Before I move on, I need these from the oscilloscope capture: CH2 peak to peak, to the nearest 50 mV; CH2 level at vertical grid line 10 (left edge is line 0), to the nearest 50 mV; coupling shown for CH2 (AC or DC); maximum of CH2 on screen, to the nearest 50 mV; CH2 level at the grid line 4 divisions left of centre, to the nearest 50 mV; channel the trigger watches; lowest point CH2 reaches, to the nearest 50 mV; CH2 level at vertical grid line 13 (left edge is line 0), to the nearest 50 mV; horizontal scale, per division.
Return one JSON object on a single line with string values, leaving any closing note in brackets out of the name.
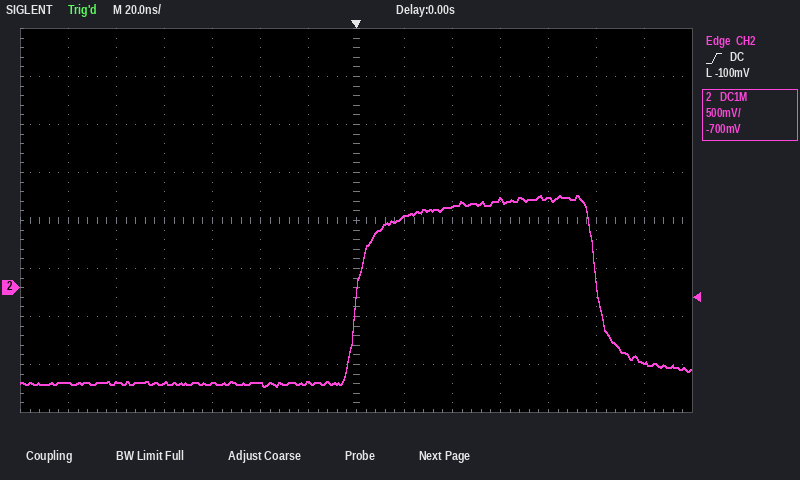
{"CH2 peak to peak, to the nearest 50 mV": "2.00 V", "CH2 level at vertical grid line 10 (left edge is line 0), to the nearest 50 mV": "900 mV", "coupling shown for CH2": "DC", "maximum of CH2 on screen, to the nearest 50 mV": "950 mV", "CH2 level at the grid line 4 divisions left of centre, to the nearest 50 mV": "-1.00 V", "channel the trigger watches": "CH2", "lowest point CH2 reaches, to the nearest 50 mV": "-1.05 V", "CH2 level at vertical grid line 13 (left edge is line 0), to the nearest 50 mV": "-800 mV", "horizontal scale, per division": "20 ns"}
